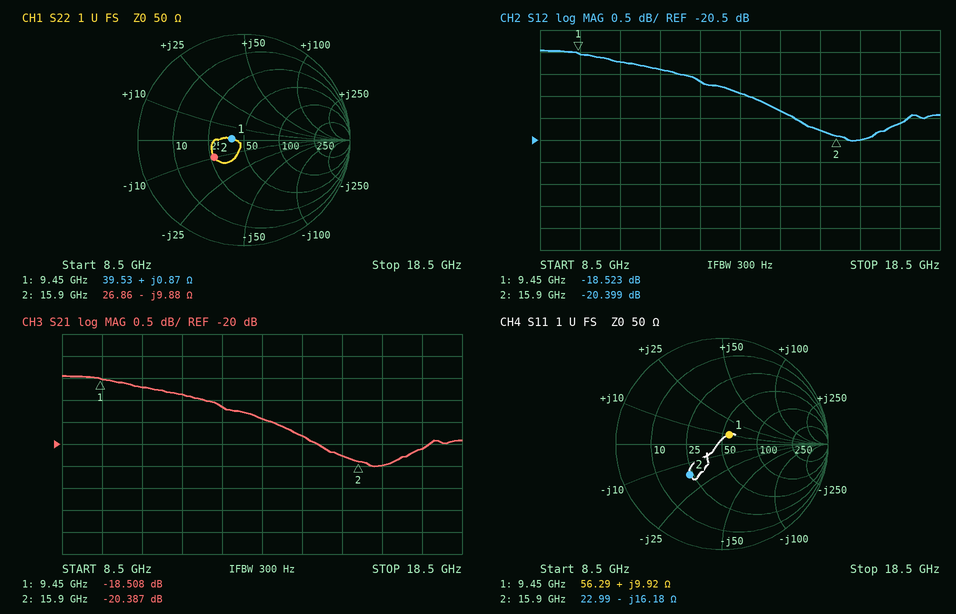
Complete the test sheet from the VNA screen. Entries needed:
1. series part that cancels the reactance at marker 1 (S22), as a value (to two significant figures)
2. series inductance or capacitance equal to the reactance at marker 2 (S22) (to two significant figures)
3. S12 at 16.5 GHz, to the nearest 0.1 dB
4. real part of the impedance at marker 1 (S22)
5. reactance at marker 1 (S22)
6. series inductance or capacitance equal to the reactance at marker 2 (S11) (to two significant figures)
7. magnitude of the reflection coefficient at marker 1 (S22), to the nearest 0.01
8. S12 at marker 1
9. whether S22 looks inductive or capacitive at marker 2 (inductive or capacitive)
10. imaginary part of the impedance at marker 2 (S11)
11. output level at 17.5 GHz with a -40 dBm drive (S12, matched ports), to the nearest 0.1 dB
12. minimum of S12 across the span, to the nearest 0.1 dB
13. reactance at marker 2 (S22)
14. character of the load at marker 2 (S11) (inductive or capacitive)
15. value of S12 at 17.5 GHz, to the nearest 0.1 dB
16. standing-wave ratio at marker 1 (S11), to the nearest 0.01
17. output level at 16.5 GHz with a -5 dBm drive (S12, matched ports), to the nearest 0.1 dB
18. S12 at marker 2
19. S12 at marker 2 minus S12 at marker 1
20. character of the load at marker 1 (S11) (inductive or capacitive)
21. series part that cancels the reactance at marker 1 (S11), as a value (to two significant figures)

19 pF
1.0 pF
-20.5 dB
39.53 Ω
+0.87 Ω
620 fF
0.12
-18.523 dB
capacitive
-16.18 Ω
-60.1 dBm
-20.5 dB
-9.88 Ω
capacitive
-20.1 dB
1.25
-25.5 dBm
-20.399 dB
-1.876 dB
inductive
1.7 pF
